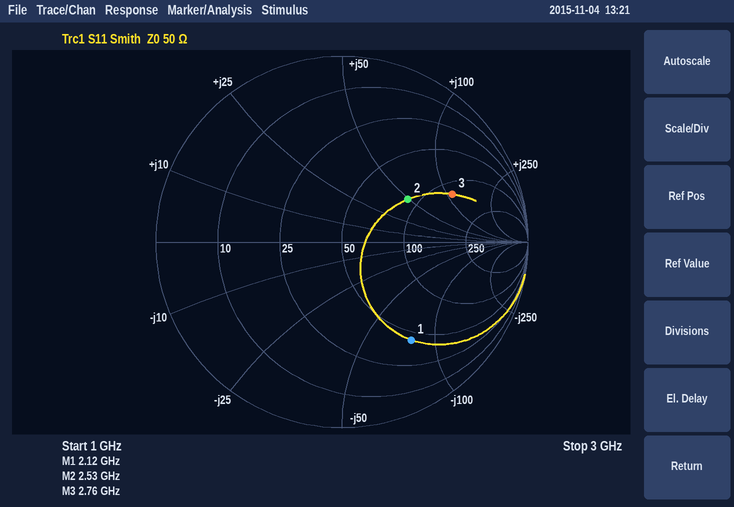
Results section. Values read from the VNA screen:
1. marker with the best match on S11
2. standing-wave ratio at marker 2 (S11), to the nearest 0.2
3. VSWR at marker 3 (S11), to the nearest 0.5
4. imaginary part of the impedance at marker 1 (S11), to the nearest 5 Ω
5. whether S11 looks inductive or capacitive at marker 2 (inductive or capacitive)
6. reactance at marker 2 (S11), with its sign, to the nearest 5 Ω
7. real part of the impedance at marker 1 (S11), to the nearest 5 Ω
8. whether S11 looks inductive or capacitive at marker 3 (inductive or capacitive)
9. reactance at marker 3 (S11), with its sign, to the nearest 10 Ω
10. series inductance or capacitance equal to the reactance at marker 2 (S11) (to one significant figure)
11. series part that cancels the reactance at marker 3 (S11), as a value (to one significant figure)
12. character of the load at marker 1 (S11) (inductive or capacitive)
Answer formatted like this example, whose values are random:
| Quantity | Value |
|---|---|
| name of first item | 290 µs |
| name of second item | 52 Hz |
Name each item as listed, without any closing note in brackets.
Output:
| Quantity | Value |
|---|---|
| marker with the best match on S11 | marker 2 |
| standing-wave ratio at marker 2 (S11), to the nearest 0.2 | 2.4 |
| VSWR at marker 3 (S11), to the nearest 0.5 | 4.5 |
| imaginary part of the impedance at marker 1 (S11), to the nearest 5 Ω | -80 Ω |
| whether S11 looks inductive or capacitive at marker 2 | inductive |
| reactance at marker 2 (S11), with its sign, to the nearest 5 Ω | +50 Ω |
| real part of the impedance at marker 1 (S11), to the nearest 5 Ω | 45 Ω |
| whether S11 looks inductive or capacitive at marker 3 | inductive |
| reactance at marker 3 (S11), with its sign, to the nearest 10 Ω | +110 Ω |
| series inductance or capacitance equal to the reactance at marker 2 (S11) | 3 nH |
| series part that cancels the reactance at marker 3 (S11), as a value | 500 fF |
| character of the load at marker 1 (S11) | capacitive |
